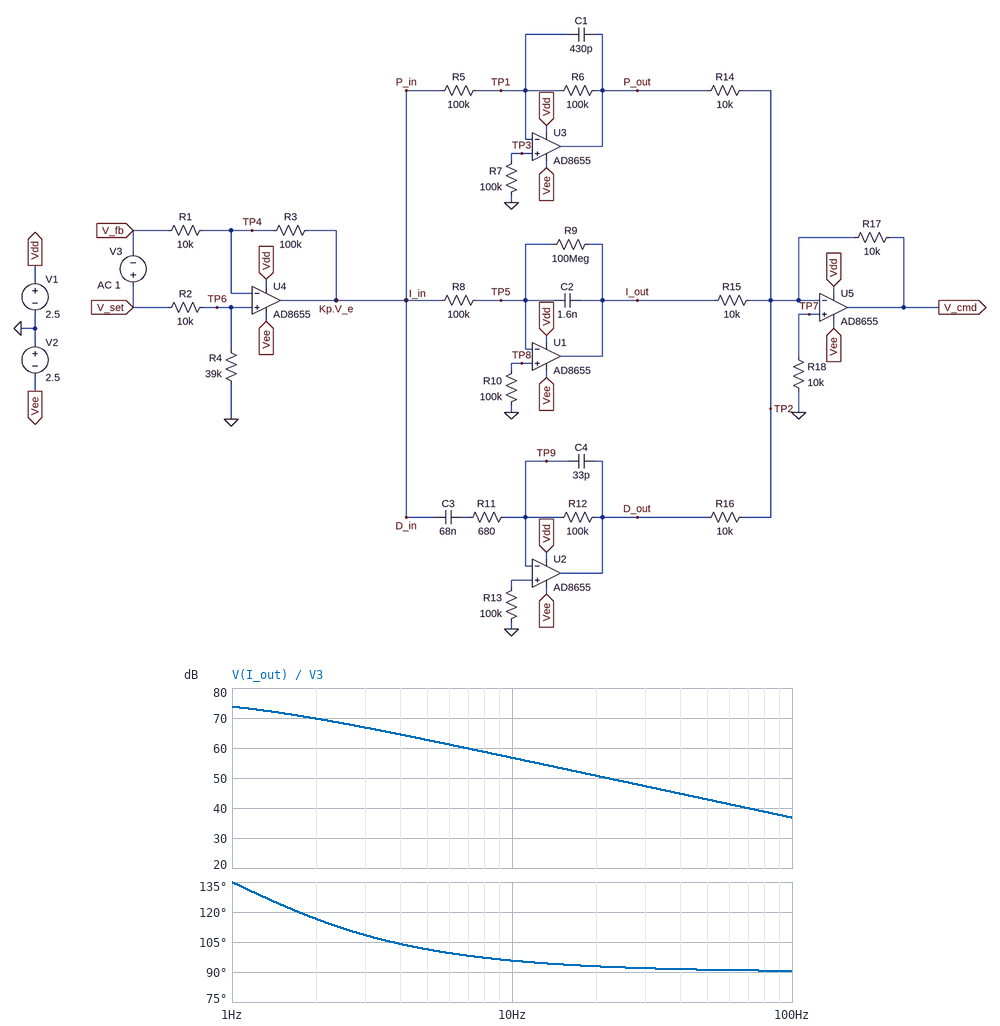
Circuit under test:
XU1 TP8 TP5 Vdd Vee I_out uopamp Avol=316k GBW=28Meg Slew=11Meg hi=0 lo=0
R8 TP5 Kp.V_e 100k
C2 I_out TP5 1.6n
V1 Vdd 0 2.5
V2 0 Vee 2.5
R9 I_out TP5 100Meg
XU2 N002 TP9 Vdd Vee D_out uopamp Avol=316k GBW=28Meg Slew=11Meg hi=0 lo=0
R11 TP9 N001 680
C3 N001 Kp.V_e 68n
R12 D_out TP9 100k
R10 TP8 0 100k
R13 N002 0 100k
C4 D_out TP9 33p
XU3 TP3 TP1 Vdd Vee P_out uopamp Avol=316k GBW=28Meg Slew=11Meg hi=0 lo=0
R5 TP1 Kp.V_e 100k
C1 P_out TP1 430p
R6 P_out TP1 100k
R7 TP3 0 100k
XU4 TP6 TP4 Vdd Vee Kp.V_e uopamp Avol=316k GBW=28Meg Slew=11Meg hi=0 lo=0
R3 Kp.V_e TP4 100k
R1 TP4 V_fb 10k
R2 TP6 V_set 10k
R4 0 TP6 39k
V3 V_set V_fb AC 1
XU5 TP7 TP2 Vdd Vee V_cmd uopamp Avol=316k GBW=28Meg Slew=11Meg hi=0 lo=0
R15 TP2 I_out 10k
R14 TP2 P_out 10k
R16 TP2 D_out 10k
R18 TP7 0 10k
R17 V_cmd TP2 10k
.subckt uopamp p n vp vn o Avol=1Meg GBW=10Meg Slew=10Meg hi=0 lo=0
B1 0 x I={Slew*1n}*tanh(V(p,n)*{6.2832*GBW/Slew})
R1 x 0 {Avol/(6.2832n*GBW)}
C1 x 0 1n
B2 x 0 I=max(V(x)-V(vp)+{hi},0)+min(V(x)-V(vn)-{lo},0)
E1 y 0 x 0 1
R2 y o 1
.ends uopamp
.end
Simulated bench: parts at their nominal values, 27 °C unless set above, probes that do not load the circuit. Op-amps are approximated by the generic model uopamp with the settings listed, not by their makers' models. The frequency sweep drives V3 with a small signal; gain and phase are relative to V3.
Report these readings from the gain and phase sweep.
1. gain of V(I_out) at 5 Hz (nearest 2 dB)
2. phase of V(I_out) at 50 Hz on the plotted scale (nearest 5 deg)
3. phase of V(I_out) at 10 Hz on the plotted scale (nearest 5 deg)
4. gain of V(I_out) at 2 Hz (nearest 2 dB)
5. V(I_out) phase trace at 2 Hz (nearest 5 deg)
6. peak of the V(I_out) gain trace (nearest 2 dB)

62 dB
90 deg
95 deg
70 dB
115 deg
74 dB
